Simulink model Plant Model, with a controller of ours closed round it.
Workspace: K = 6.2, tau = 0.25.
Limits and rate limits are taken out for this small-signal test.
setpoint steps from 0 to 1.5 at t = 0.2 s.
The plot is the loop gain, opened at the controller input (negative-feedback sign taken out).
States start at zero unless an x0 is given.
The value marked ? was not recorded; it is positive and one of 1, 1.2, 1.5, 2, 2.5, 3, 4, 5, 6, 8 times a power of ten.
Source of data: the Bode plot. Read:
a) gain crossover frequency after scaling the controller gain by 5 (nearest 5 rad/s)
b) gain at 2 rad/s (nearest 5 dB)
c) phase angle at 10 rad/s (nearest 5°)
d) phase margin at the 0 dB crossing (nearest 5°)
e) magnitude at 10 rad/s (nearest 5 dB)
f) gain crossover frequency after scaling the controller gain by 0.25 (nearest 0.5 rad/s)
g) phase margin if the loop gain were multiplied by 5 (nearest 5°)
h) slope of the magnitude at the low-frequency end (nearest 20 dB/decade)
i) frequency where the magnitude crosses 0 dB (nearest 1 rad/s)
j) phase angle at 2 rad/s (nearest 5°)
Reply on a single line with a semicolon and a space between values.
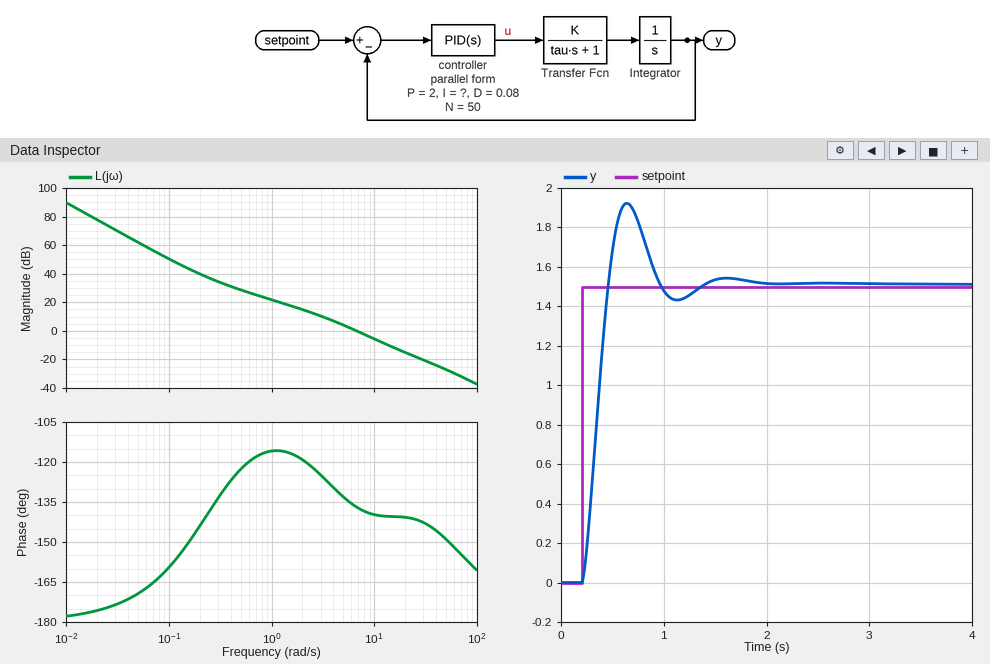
20 rad/s; 15 dB; -140°; 45°; -5 dB; 2.5 rad/s; 40°; -40 dB/decade; 7 rad/s; -120°
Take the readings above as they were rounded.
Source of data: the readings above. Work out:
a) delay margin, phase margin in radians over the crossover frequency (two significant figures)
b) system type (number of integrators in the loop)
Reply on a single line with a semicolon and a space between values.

0.11 s; 2
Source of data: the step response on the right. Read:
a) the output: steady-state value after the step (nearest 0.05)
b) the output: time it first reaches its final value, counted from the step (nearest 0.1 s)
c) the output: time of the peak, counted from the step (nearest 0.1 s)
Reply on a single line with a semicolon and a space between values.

1.50; 0.3 s; 0.4 s
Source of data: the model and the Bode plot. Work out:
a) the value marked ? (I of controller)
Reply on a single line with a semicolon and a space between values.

0.5
